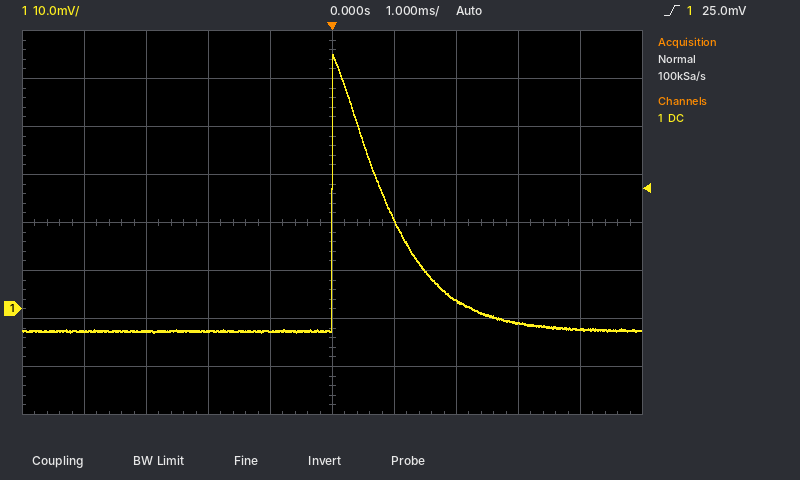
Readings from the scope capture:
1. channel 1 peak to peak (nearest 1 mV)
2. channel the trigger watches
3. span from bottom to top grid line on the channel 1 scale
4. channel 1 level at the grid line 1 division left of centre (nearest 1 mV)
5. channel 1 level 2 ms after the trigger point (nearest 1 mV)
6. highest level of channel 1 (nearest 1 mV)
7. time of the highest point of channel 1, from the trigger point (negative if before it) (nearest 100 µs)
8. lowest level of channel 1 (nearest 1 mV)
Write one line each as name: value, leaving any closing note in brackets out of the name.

channel 1 peak to peak: 58 mV
channel the trigger watches: channel 1
span from bottom to top grid line on the channel 1 scale: 80 mV
channel 1 level at the grid line 1 division left of centre: -5 mV
channel 1 level 2 ms after the trigger point: 2 mV
highest level of channel 1: 53 mV
time of the highest point of channel 1, from the trigger point (negative if before it): 0.0 ms
lowest level of channel 1: -5 mV
